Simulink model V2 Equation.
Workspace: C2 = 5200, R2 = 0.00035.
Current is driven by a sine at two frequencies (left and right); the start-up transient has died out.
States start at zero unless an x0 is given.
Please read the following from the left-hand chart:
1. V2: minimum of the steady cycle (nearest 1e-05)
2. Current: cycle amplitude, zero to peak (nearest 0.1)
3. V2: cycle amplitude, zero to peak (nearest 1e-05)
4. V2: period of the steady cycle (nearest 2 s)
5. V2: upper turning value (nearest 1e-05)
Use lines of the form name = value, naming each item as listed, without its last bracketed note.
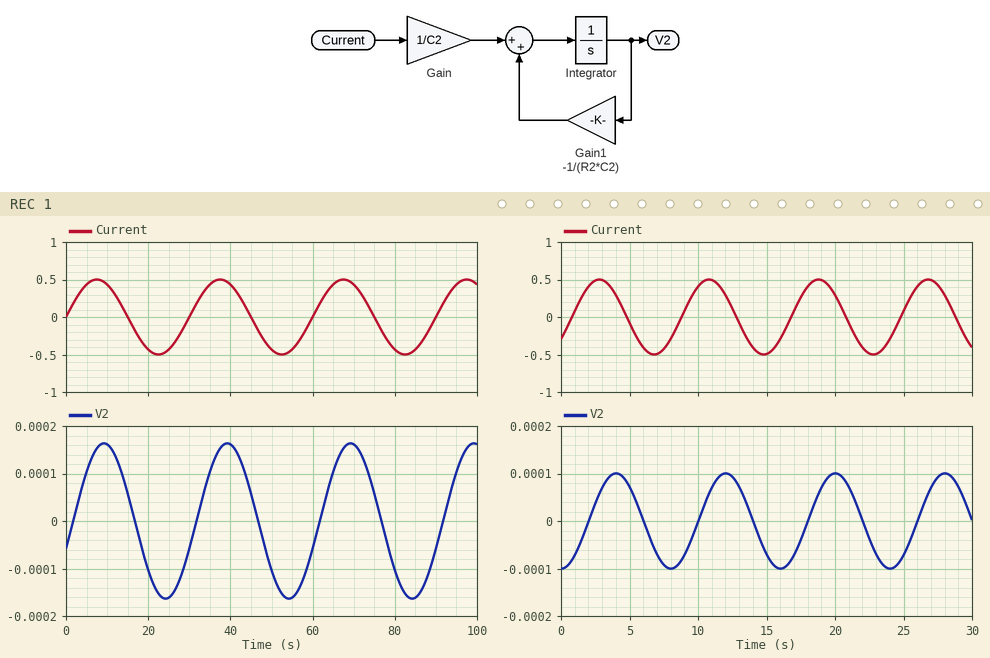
V2: minimum of the steady cycle = -0.00016
Current: cycle amplitude, zero to peak = 0.5
V2: cycle amplitude, zero to peak = 0.00016
V2: period of the steady cycle = 30 s
V2: upper turning value = 0.00016
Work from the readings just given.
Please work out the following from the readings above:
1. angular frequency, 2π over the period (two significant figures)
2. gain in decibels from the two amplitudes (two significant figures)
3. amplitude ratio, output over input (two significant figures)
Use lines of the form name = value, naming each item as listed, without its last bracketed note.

angular frequency, 2π over the period = 0.21 rad/s
gain in decibels from the two amplitudes = -70 dB
amplitude ratio, output over input = 0.00032
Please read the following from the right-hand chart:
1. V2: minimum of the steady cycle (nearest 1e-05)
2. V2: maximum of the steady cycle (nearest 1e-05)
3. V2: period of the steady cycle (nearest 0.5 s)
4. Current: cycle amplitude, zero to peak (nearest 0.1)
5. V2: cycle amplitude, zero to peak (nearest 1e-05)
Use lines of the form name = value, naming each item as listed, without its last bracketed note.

V2: minimum of the steady cycle = -0.00010
V2: maximum of the steady cycle = 0.00010
V2: period of the steady cycle = 8.0 s
Current: cycle amplitude, zero to peak = 0.5
V2: cycle amplitude, zero to peak = 0.00010
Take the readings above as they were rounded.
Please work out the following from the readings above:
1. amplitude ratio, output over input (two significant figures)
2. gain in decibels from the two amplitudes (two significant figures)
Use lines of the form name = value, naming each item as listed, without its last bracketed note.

amplitude ratio, output over input = 0.00020
gain in decibels from the two amplitudes = -74 dB
